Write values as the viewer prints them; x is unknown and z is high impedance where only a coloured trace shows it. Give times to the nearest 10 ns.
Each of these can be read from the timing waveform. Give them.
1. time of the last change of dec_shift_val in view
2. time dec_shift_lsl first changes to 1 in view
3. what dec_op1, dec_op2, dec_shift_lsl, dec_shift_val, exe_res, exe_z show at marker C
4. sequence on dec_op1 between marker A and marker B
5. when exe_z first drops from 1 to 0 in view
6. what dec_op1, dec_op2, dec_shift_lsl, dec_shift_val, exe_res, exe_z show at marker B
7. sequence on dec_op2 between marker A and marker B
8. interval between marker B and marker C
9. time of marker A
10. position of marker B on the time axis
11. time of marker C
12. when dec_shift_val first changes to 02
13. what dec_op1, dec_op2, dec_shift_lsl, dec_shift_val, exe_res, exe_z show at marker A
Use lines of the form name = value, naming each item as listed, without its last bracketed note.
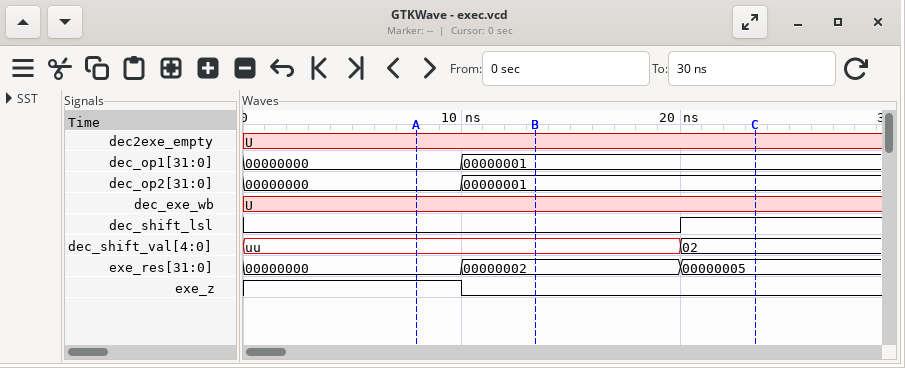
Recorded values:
time of the last change of dec_shift_val in view = 20 ns
time dec_shift_lsl first changes to 1 in view = 20 ns
what dec_op1, dec_op2, dec_shift_lsl, dec_shift_val, exe_res, exe_z show at marker C = dec_op1=00000001, dec_op2=00000001, dec_shift_lsl=1, dec_shift_val=02, exe_res=00000005, exe_z=0
sequence on dec_op1 between marker A and marker B = 00000000, 00000001
when exe_z first drops from 1 to 0 in view = 10 ns
what dec_op1, dec_op2, dec_shift_lsl, dec_shift_val, exe_res, exe_z show at marker B = dec_op1=00000001, dec_op2=00000001, dec_shift_lsl=0, dec_shift_val=uu, exe_res=00000002, exe_z=0
sequence on dec_op2 between marker A and marker B = 00000000, 00000001
interval between marker B and marker C = 10 ns
time of marker A = 10 ns
position of marker B on the time axis = 10 ns
time of marker C = 20 ns
when dec_shift_val first changes to 02 = 20 ns
what dec_op1, dec_op2, dec_shift_lsl, dec_shift_val, exe_res, exe_z show at marker A = dec_op1=00000000, dec_op2=00000000, dec_shift_lsl=0, dec_shift_val=uu, exe_res=00000000, exe_z=1
